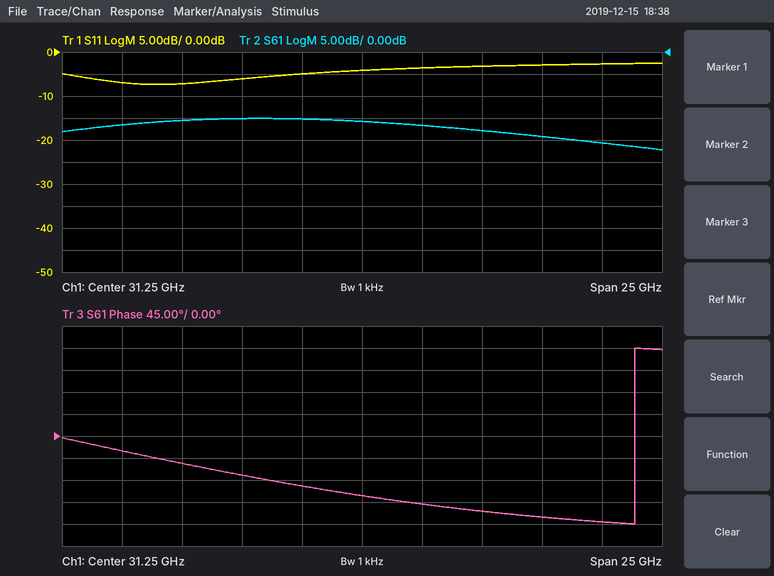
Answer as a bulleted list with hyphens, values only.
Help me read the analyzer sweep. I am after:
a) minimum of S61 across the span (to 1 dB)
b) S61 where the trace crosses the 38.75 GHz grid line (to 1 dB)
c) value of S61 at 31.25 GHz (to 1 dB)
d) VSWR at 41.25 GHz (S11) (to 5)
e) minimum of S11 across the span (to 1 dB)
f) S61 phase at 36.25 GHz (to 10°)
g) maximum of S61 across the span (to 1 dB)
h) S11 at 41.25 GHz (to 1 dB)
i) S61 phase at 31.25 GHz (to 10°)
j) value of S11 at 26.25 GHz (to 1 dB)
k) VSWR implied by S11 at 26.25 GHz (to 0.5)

- -22 dB
- -19 dB
- -16 dB
- 5
- -7 dB
- -150°
- -15 dB
- -3 dB
- -120°
- -6 dB
- 3.0
